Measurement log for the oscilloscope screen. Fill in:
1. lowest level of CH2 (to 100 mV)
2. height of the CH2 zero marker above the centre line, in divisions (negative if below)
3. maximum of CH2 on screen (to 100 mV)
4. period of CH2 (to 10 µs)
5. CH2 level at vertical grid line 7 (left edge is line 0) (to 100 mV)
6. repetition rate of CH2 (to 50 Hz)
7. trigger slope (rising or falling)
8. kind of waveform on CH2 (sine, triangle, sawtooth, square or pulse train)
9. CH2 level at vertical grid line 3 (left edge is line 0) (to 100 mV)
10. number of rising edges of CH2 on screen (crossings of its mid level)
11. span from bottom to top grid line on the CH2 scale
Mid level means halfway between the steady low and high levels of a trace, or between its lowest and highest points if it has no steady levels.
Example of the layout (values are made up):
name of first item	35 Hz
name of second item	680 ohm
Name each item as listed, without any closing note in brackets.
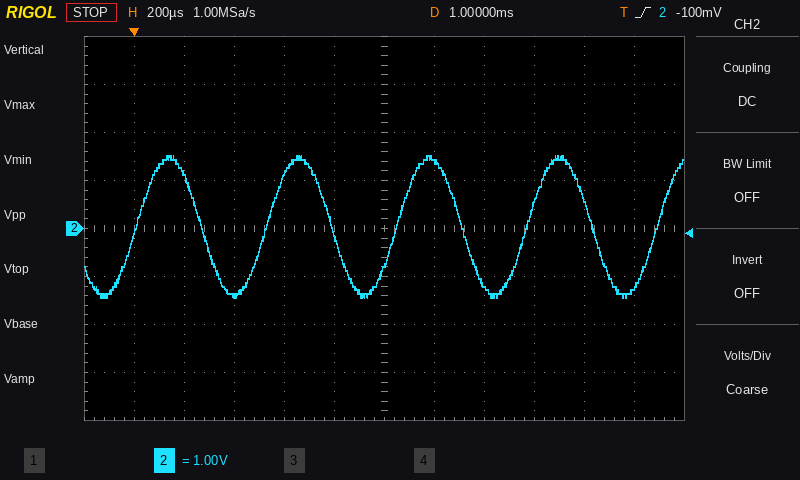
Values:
lowest level of CH2	-1.4 V
height of the CH2 zero marker above the centre line, in divisions	0.0 div
maximum of CH2 on screen	1.5 V
period of CH2	520 µs
CH2 level at vertical grid line 7 (left edge is line 0)	1.4 V
repetition rate of CH2	1.90 kHz
trigger slope	rising
kind of waveform on CH2	sine
CH2 level at vertical grid line 3 (left edge is line 0)	-1.4 V
number of rising edges of CH2 on screen	5
span from bottom to top grid line on the CH2 scale	8 V
